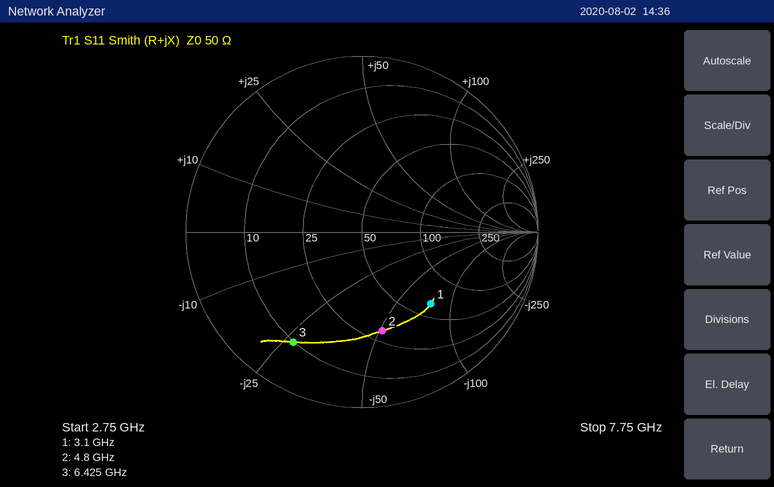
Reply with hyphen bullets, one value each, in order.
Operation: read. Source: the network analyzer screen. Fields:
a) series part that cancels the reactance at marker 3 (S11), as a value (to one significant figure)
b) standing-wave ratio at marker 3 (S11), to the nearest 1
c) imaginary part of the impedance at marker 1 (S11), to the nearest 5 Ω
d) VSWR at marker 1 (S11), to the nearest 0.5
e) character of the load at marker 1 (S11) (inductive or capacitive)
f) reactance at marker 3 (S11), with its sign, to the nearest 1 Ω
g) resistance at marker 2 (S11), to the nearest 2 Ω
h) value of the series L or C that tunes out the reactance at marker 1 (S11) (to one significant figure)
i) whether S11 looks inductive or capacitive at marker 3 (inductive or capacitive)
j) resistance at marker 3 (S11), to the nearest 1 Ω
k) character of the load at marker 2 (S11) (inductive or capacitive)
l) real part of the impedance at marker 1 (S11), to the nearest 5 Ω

- 700 pH
- 7
- -75 Ω
- 3.5
- capacitive
- -27 Ω
- 30 Ω
- 4 nH
- capacitive
- 10 Ω
- capacitive
- 65 Ω
